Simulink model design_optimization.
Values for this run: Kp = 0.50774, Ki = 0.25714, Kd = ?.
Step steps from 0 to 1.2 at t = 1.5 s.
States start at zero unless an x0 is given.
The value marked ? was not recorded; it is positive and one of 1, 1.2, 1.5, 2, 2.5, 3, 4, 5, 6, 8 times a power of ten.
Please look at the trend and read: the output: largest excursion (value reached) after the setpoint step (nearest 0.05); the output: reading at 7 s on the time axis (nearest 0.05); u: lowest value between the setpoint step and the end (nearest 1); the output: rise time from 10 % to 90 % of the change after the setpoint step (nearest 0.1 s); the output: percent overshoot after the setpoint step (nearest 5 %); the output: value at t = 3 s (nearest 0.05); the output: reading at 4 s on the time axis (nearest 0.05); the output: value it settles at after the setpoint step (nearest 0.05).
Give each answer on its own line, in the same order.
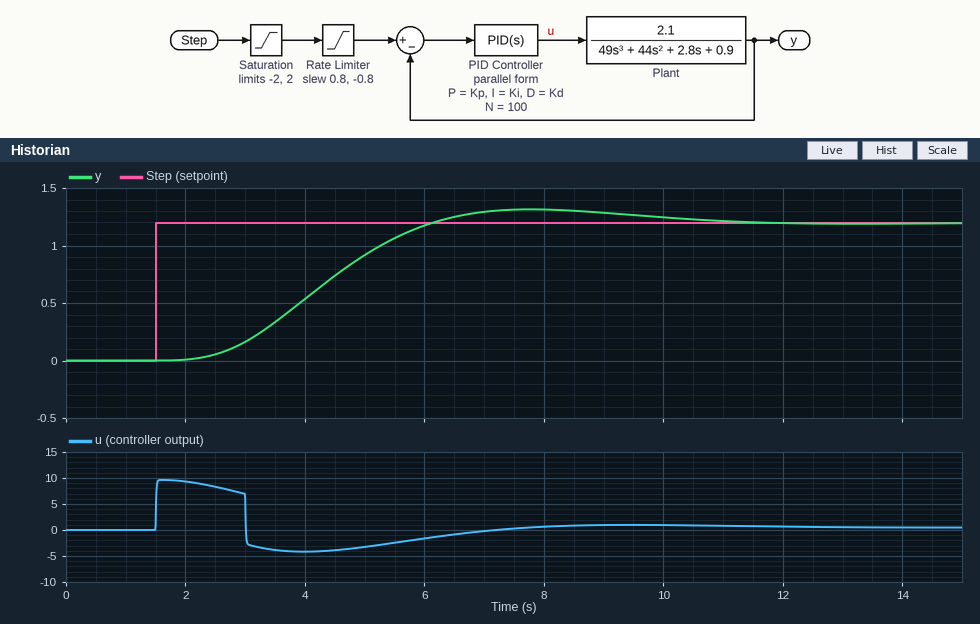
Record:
1.30
1.30
-4
2.7 s
10 %
0.15
0.55
1.20
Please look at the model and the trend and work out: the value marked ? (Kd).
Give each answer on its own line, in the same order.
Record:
12
